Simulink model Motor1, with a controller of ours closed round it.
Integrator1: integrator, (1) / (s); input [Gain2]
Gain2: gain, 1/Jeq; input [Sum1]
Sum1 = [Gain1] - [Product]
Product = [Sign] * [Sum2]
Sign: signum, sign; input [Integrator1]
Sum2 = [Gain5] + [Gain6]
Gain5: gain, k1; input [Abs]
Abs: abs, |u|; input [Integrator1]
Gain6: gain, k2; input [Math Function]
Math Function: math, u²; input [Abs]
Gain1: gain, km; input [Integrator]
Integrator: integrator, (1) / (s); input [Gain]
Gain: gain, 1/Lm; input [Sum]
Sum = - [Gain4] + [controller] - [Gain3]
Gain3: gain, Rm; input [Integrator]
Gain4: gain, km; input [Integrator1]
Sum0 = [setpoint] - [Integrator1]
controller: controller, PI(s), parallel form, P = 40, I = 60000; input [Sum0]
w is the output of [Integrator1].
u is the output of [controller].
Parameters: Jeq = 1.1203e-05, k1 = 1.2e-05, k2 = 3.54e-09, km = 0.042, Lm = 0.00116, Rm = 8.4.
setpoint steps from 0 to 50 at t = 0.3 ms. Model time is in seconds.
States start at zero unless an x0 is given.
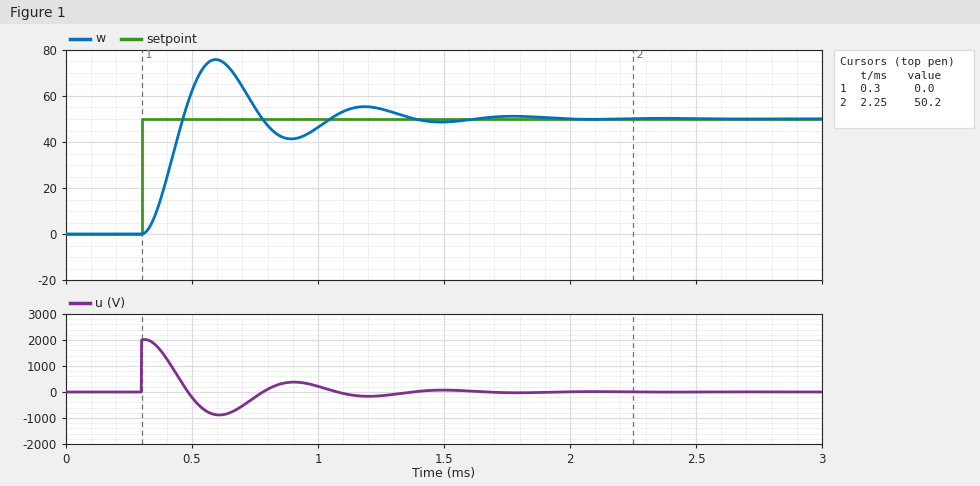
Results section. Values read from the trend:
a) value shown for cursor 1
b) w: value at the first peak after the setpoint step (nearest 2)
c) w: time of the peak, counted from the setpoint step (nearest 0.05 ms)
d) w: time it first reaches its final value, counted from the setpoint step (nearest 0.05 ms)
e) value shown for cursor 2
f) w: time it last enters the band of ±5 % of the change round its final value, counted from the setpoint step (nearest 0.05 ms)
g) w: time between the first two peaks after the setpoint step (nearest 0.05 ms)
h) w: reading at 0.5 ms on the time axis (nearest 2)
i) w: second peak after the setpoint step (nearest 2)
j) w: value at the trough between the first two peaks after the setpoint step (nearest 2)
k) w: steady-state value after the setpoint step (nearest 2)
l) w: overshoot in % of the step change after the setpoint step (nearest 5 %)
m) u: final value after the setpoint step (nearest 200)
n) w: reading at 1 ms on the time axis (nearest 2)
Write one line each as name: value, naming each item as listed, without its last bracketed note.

value shown for cursor 1: 0.0
w: value at the first peak after the setpoint step: 76
w: time of the peak, counted from the setpoint step: 0.30 ms
w: time it first reaches its final value, counted from the setpoint step: 0.15 ms
value shown for cursor 2: 50.2
w: time it last enters the band of ±5 % of the change round its final value, counted from the setpoint step: 1.00 ms
w: time between the first two peaks after the setpoint step: 0.60 ms
w: reading at 0.5 ms on the time axis: 62
w: second peak after the setpoint step: 56
w: value at the trough between the first two peaks after the setpoint step: 42
w: steady-state value after the setpoint step: 50
w: overshoot in % of the step change after the setpoint step: 50 %
u: final value after the setpoint step: 0
w: reading at 1 ms on the time axis: 46
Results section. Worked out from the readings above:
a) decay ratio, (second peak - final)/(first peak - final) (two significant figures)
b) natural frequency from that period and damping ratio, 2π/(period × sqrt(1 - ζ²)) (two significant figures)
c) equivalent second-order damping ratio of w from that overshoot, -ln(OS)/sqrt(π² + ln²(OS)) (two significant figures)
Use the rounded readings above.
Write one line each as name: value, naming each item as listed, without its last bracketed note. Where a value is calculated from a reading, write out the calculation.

decay ratio, (second peak - final)/(first peak - final): (56 - 50) / (76 - 50) = 0.23
natural frequency from that period and damping ratio, 2π/(period × sqrt(1 - ζ²)): 2π / (0.6 × sqrt(1 - 0.22²)) = 11 rad/ms
equivalent second-order damping ratio of w from that overshoot, -ln(OS)/sqrt(π² + ln²(OS)): ln(0.5) = -0.693; 0.693 / sqrt(9.870 + 0.480) = 0.22
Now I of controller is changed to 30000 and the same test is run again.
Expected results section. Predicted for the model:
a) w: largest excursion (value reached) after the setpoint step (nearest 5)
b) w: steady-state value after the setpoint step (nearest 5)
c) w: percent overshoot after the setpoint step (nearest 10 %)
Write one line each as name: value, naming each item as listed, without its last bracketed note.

w: largest excursion (value reached) after the setpoint step: 70
w: steady-state value after the setpoint step: 50
w: percent overshoot after the setpoint step: 40 %
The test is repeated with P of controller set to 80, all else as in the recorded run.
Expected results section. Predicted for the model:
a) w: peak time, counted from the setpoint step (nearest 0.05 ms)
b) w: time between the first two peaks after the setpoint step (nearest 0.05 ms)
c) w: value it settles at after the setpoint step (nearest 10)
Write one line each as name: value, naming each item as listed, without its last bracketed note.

w: peak time, counted from the setpoint step: 0.20 ms
w: time between the first two peaks after the setpoint step: 0.40 ms
w: value it settles at after the setpoint step: 50
